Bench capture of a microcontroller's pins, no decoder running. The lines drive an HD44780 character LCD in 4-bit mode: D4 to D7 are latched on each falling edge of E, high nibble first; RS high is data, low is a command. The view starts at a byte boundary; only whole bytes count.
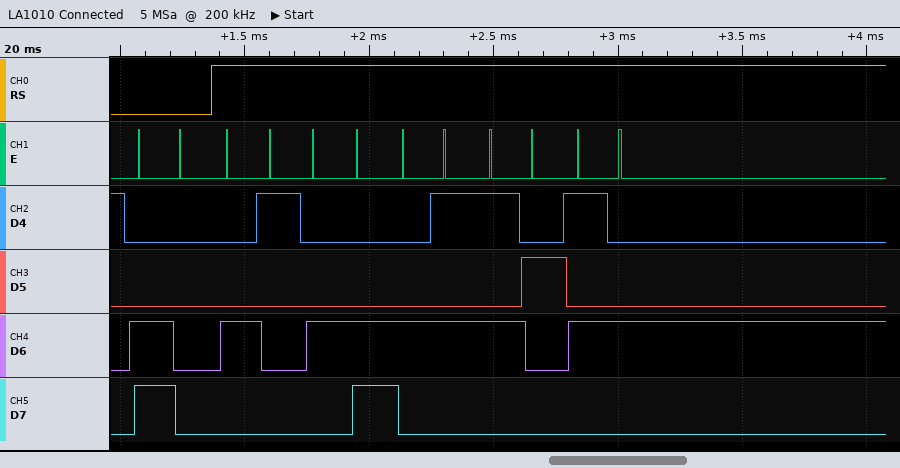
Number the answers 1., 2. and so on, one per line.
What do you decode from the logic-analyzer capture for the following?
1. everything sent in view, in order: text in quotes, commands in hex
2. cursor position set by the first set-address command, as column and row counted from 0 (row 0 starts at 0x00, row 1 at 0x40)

1. 0xC0 "ALERT"
2. column 0, row 1
